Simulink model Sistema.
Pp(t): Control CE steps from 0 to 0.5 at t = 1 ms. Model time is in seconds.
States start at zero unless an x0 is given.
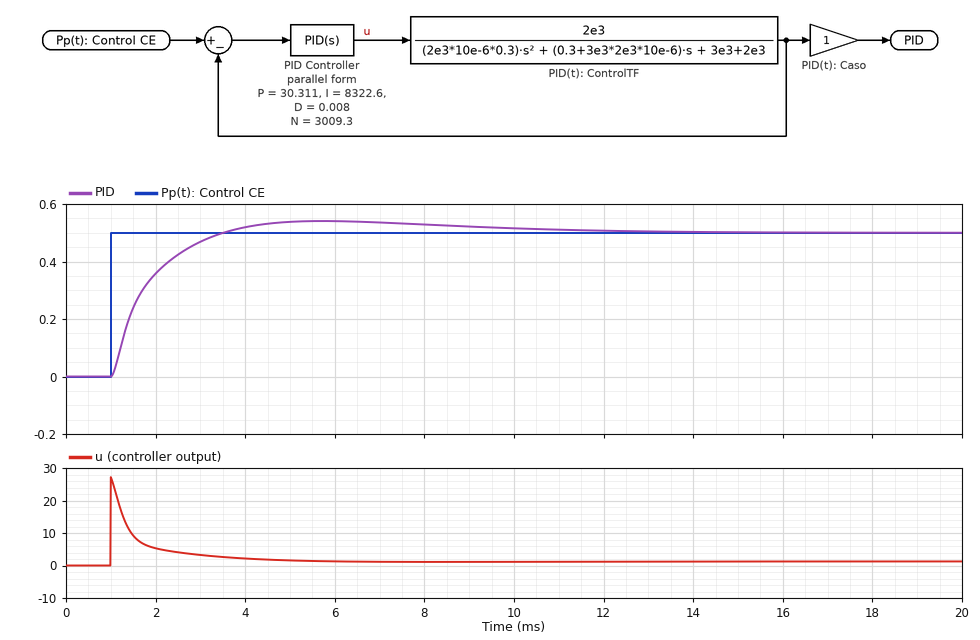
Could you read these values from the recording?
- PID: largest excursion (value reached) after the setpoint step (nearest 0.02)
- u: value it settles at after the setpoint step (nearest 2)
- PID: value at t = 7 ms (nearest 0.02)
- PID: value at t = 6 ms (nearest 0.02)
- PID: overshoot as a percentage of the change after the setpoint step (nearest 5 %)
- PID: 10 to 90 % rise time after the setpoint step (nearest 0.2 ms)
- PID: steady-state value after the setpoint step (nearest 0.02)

0.54
2
0.54
0.54
10 %
1.6 ms
0.50
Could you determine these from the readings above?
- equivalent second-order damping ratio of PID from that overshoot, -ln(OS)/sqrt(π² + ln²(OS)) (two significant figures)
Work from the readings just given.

0.59
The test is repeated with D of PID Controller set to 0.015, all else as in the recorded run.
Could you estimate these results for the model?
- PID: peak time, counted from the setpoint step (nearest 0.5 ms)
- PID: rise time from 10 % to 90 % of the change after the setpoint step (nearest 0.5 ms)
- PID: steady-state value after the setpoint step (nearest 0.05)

5.5 ms
2.0 ms
0.50
